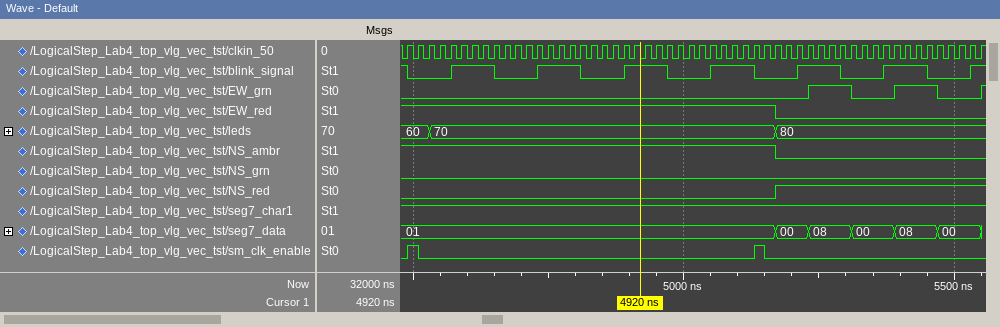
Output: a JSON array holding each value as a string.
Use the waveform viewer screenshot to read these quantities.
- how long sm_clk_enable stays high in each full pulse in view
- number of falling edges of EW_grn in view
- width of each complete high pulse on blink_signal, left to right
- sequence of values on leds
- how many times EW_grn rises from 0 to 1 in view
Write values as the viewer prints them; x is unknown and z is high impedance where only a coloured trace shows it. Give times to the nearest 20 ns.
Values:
["20 ns, 20 ns", "2", "80 ns, 80 ns, 80 ns, 80 ns, 80 ns, 80 ns", "60, 70, 80", "3"]
